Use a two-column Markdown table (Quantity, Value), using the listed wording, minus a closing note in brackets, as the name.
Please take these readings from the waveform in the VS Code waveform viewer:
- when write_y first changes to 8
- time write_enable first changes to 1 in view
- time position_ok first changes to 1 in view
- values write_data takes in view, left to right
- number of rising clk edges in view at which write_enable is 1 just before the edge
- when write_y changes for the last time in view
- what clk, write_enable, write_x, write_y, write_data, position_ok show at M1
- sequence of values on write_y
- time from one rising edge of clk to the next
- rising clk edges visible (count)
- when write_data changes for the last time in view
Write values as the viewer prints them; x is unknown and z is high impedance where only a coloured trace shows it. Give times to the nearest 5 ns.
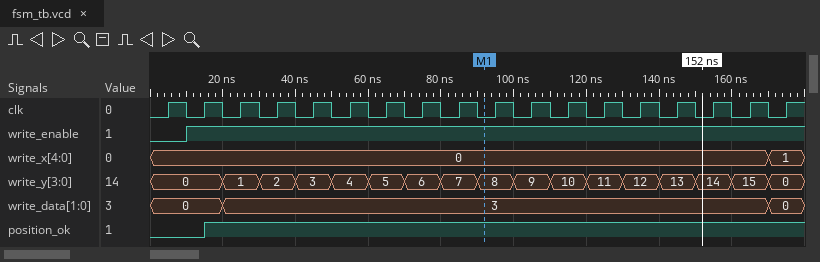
| Quantity | Value |
|---|---|
| when write_y first changes to 8 | 90 ns |
| time write_enable first changes to 1 in view | 10 ns |
| time position_ok first changes to 1 in view | 15 ns |
| values write_data takes in view, left to right | 0, 3, 0 |
| number of rising clk edges in view at which write_enable is 1 just before the edge | 17 |
| when write_y changes for the last time in view | 170 ns |
| what clk, write_enable, write_x, write_y, write_data, position_ok show at M1 | clk=0, write_enable=1, write_x=0, write_y=8, write_data=3, position_ok=1 |
| sequence of values on write_y | 0, 1, 2, 3, 4, 5, 6, 7, 8, 9, 10, 11, 12, 13, 14, 15, 0 |
| time from one rising edge of clk to the next | 10 ns |
| rising clk edges visible | 18 |
| when write_data changes for the last time in view | 170 ns |
